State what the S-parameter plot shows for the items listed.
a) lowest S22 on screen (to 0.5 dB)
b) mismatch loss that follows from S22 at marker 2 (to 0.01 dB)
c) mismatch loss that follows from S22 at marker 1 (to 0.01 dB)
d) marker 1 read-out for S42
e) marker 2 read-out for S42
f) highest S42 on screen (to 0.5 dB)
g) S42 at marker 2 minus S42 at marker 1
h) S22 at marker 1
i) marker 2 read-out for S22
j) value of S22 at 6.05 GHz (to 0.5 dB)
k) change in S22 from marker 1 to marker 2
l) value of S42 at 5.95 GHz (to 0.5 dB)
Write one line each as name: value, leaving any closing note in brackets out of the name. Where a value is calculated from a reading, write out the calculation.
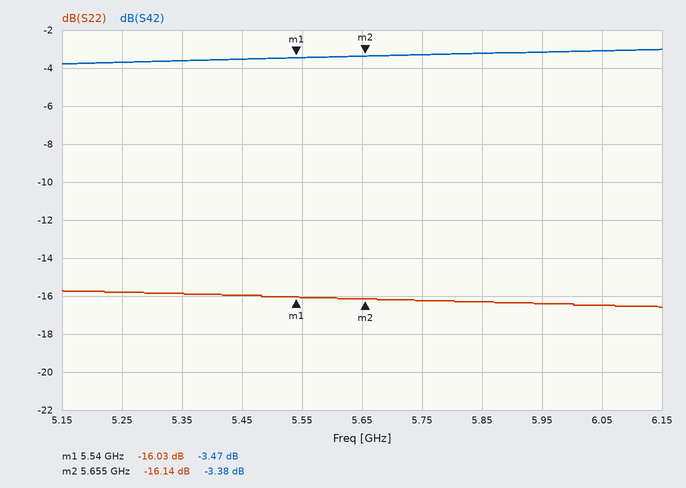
lowest S22 on screen: -16.5 dB
mismatch loss that follows from S22 at marker 2: −10 log10(1 − 10^(-16.14/10)) ≈ 0.11 dB
mismatch loss that follows from S22 at marker 1: −10 log10(1 − 10^(-16.03/10)) ≈ 0.11 dB
marker 1 read-out for S42: -3.47 dB
marker 2 read-out for S42: -3.38 dB
highest S42 on screen: -3.0 dB
S42 at marker 2 minus S42 at marker 1: -3.38 − (-3.47) = 0.09 dB
S22 at marker 1: -16.03 dB
marker 2 read-out for S22: -16.14 dB
value of S22 at 6.05 GHz: -16.5 dB
change in S22 from marker 1 to marker 2: -16.14 − (-16.03) = -0.11 dB
value of S42 at 5.95 GHz: -3.0 dB
